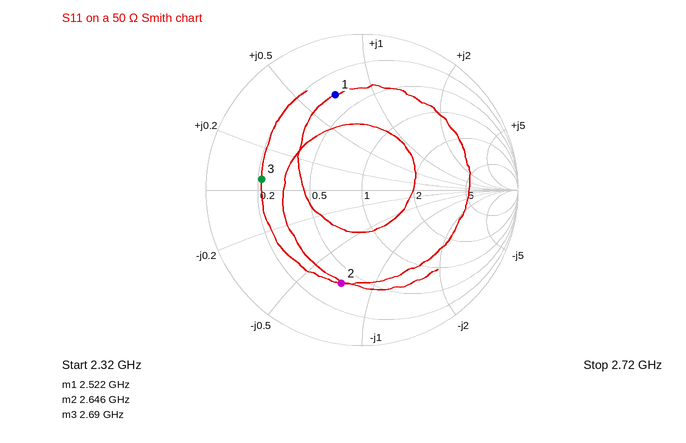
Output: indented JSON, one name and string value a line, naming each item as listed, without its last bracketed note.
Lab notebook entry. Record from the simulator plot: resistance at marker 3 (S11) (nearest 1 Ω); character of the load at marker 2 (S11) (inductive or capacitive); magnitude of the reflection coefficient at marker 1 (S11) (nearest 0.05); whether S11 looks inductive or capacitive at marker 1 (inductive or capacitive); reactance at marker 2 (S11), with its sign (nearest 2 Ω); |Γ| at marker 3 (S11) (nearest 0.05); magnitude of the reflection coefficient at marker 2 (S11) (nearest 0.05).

{
  "resistance at marker 3 (S11)": "11 Ω",
  "character of the load at marker 2 (S11)": "capacitive",
  "magnitude of the reflection coefficient at marker 1 (S11)": "0.65",
  "whether S11 looks inductive or capacitive at marker 1": "inductive",
  "reactance at marker 2 (S11), with its sign": "-36 Ω",
  "|Γ| at marker 3 (S11)": "0.65",
  "magnitude of the reflection coefficient at marker 2 (S11)": "0.60"
}
